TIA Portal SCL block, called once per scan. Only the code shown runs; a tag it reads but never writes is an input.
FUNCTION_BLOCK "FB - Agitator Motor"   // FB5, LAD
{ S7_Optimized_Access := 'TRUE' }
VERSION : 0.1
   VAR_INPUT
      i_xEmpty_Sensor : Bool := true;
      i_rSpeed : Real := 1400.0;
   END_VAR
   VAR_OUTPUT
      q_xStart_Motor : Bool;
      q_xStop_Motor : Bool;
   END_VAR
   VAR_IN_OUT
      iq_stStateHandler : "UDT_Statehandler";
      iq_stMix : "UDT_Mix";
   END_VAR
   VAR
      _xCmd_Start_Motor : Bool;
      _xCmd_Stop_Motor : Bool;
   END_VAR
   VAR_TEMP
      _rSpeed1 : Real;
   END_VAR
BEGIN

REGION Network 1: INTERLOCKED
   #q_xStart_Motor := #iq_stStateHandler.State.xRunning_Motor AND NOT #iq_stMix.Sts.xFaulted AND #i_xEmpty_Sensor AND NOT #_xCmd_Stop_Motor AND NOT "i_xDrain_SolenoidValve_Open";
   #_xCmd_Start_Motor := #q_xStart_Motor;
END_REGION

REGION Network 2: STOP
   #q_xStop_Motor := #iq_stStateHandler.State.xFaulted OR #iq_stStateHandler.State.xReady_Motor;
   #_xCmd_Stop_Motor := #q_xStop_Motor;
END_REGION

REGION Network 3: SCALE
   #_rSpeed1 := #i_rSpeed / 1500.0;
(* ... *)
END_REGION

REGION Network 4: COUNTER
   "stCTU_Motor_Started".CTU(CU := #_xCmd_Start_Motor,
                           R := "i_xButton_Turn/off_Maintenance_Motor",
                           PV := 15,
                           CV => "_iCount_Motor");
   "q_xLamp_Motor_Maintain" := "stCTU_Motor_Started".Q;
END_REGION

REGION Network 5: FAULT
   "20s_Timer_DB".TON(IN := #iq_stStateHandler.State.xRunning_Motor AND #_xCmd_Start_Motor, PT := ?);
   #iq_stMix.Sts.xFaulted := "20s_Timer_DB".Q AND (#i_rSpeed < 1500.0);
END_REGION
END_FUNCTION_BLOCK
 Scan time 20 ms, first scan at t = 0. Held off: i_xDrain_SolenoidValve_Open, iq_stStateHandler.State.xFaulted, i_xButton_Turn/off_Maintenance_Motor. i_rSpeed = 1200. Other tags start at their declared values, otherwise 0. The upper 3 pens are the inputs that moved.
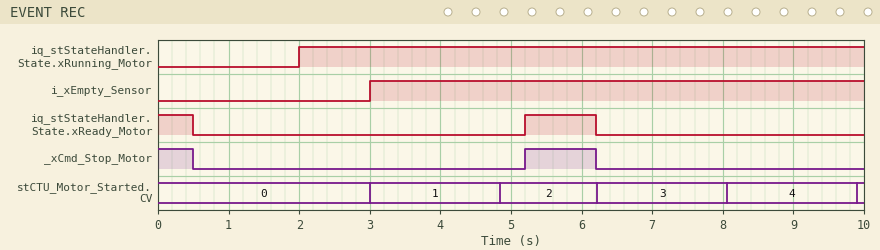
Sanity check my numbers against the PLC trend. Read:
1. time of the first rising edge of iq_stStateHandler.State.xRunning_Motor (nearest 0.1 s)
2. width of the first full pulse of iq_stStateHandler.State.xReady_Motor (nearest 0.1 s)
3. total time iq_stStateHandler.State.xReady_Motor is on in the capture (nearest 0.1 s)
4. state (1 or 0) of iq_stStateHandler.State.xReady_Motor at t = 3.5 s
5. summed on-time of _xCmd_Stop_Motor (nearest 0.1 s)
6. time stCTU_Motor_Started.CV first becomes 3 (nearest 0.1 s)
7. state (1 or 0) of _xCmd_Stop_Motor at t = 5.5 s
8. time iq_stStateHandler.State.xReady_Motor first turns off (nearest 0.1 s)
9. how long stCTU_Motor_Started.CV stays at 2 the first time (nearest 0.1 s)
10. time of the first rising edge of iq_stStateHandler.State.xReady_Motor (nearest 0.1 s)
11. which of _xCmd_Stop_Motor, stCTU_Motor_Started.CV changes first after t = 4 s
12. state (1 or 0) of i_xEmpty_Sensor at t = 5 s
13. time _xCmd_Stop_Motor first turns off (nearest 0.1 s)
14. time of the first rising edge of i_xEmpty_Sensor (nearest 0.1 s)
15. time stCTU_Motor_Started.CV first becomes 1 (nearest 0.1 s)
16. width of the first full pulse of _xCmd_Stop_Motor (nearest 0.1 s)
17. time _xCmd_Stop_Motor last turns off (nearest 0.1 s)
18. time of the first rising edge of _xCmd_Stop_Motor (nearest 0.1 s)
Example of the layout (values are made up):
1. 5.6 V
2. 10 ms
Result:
1. 2.0 s
2. 1.0 s
3. 1.5 s
4. 0
5. 1.5 s
6. 6.2 s
7. 1
8. 0.5 s
9. 1.4 s
10. 5.2 s
11. stCTU_Motor_Started.CV
12. 1
13. 0.5 s
14. 3.0 s
15. 3.0 s
16. 1.0 s
17. 6.2 s
18. 5.2 s
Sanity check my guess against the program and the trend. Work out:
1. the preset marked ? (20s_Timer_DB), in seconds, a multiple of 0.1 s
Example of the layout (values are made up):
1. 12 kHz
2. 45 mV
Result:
1. 1.8 s
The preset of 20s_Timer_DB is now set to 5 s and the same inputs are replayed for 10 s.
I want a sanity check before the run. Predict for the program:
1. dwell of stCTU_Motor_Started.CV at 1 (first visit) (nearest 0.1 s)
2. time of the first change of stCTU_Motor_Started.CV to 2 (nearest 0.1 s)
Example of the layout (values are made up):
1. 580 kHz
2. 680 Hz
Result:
1. 3.2 s
2. 6.2 s
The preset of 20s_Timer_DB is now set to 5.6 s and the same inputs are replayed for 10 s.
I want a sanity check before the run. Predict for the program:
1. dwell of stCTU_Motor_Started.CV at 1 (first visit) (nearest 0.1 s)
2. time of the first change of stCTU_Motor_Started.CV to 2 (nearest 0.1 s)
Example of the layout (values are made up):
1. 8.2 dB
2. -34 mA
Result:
1. 3.2 s
2. 6.2 s
